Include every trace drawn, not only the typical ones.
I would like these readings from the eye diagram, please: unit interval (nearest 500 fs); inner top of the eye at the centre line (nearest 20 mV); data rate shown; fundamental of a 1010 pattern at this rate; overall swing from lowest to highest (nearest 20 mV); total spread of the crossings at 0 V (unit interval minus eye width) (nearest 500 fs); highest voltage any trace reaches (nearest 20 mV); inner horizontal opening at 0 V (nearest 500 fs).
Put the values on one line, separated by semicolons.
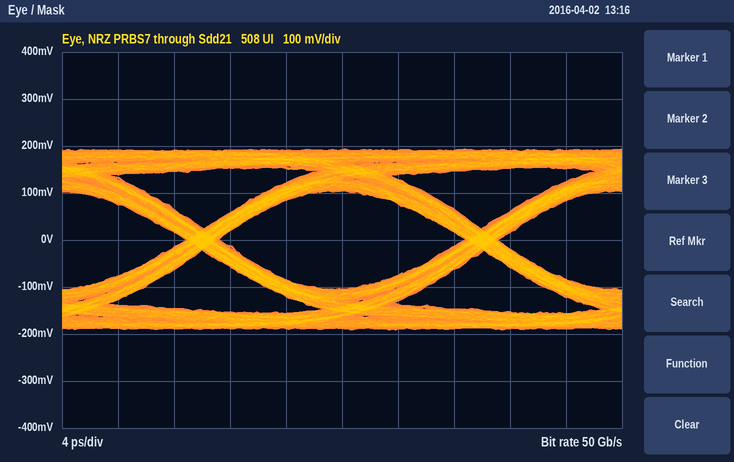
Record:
20.0 ps; 100 mV; 50 Gb/s; 25 GHz; 380 mV; 2.5 ps; 200 mV; 17.5 ps
